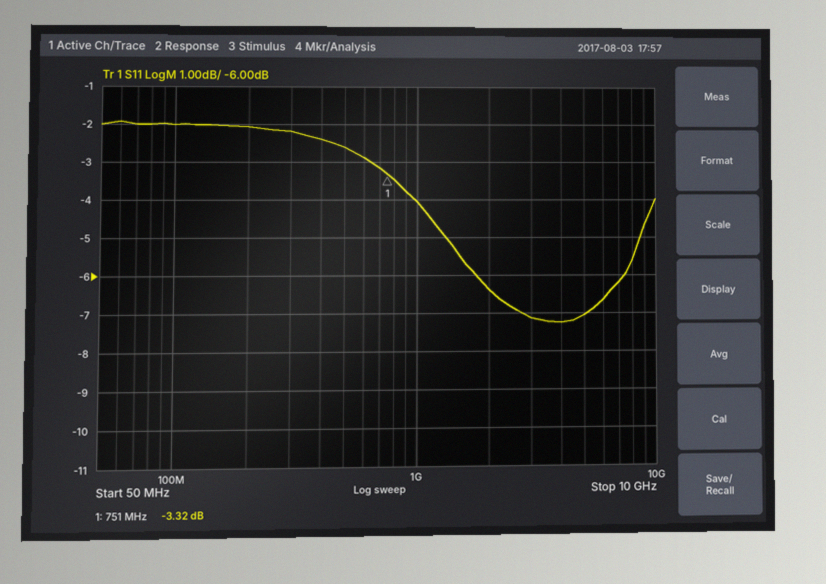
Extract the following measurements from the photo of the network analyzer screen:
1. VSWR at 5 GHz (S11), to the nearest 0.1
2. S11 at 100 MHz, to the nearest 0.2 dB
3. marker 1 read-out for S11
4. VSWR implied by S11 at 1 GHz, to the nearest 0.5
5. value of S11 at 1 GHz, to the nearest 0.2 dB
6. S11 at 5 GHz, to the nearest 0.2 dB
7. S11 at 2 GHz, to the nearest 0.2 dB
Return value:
2.6
-2.0 dB
-3.32 dB
4.5
-4.0 dB
-7.0 dB
-6.4 dB
